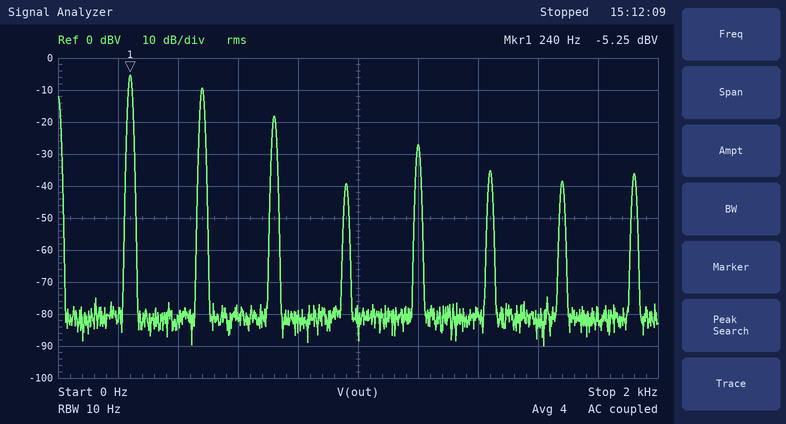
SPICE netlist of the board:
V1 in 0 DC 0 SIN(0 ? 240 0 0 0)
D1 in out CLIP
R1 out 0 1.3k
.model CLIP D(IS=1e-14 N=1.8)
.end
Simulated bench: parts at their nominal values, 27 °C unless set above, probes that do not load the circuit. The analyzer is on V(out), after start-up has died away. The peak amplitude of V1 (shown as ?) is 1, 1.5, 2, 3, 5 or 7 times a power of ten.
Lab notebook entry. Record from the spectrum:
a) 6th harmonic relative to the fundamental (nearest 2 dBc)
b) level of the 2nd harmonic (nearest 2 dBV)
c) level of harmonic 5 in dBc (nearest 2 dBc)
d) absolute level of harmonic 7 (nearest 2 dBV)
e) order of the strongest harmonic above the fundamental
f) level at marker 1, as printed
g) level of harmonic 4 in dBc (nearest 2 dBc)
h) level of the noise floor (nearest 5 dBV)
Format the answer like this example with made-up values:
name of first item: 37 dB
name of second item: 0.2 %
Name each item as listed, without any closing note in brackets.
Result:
6th harmonic relative to the fundamental: -30 dBc
level of the 2nd harmonic: -10 dBV
level of harmonic 5 in dBc: -22 dBc
absolute level of harmonic 7: -38 dBV
order of the strongest harmonic above the fundamental: 2
level at marker 1, as printed: -5.25 dBV
level of harmonic 4 in dBc: -34 dBc
level of the noise floor: -80 dBV
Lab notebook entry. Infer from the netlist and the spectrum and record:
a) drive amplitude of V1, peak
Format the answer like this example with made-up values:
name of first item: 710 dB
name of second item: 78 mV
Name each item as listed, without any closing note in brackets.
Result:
drive amplitude of V1, peak: 3 V
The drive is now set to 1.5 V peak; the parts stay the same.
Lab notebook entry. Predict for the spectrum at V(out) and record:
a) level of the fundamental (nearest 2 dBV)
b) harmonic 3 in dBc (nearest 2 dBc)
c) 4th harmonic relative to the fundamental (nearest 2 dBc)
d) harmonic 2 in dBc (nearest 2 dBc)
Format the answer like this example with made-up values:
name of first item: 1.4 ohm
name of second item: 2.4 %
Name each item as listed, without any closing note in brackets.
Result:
level of the fundamental: -22 dBV
harmonic 3 in dBc: -6 dBc
4th harmonic relative to the fundamental: -10 dBc
harmonic 2 in dBc: -2 dBc
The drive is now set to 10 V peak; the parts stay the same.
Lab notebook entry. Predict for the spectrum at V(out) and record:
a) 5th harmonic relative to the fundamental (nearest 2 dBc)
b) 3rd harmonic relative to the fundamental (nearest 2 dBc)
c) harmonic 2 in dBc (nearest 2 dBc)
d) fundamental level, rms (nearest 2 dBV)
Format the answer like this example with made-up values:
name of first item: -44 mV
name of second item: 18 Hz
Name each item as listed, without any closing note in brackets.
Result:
5th harmonic relative to the fundamental: -30 dBc
3rd harmonic relative to the fundamental: -24 dBc
harmonic 2 in dBc: -6 dBc
fundamental level, rms: 10 dBV
